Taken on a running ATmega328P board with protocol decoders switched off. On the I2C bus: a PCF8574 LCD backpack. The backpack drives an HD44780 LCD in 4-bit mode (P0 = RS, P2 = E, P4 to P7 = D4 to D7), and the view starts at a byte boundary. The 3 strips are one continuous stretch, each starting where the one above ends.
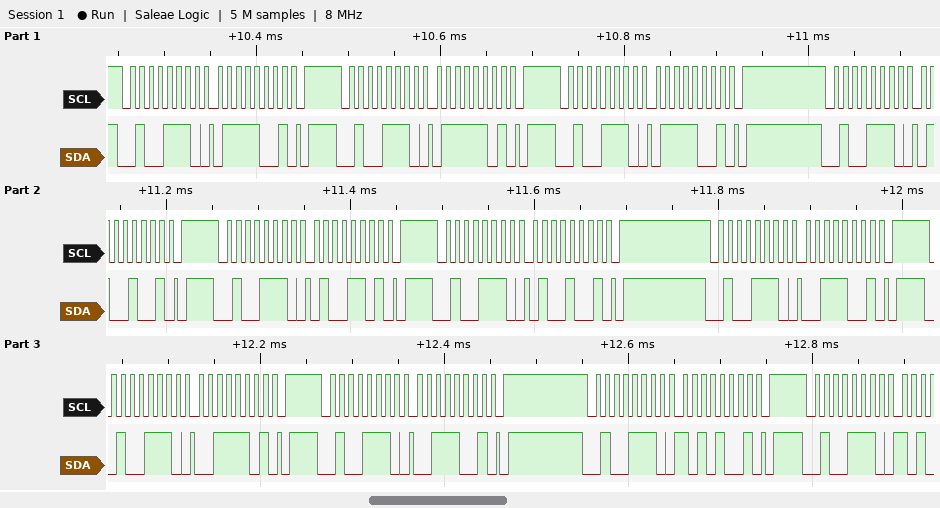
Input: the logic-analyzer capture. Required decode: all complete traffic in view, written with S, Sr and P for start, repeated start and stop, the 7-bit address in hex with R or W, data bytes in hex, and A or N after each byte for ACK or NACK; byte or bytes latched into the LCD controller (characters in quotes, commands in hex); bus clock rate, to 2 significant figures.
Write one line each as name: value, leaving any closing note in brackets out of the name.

all complete traffic in view, written with S, Sr and P for start, repeated start and stop, the 7-bit address in hex with R or W, data bytes in hex, and A or N after each byte for ACK or NACK: S 27W A 79 A P S 27W A 7D A P S 27W A 79 A P S 27W A 49 A P S 27W A 4D A P S 27W A 49 A P S 27W A 39 A P S 27W A 3D A P S 27W A 39 A P S 27W A A9 A P S 27W A
byte or bytes latched into the LCD controller: 't'
bus clock rate, to 2 significant figures: 100 kHz
